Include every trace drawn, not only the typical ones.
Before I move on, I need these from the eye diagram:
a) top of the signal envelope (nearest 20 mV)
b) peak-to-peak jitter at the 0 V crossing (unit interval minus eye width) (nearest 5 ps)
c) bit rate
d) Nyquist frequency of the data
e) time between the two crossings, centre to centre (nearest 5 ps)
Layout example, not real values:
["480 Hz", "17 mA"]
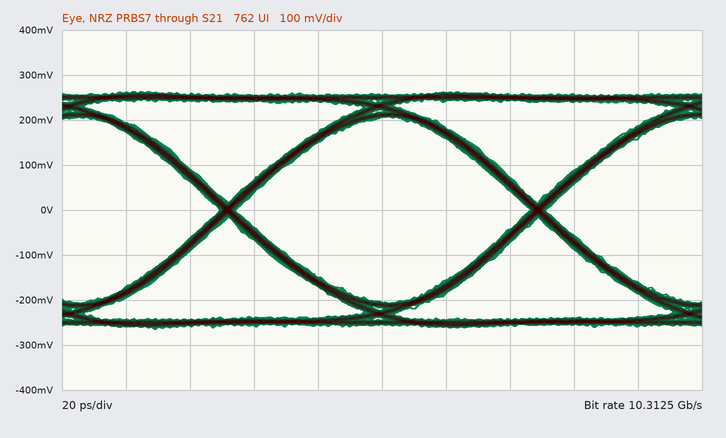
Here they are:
["260 mV", "5 ps", "10.3125 Gb/s", "5.15625 GHz", "95 ps"]
